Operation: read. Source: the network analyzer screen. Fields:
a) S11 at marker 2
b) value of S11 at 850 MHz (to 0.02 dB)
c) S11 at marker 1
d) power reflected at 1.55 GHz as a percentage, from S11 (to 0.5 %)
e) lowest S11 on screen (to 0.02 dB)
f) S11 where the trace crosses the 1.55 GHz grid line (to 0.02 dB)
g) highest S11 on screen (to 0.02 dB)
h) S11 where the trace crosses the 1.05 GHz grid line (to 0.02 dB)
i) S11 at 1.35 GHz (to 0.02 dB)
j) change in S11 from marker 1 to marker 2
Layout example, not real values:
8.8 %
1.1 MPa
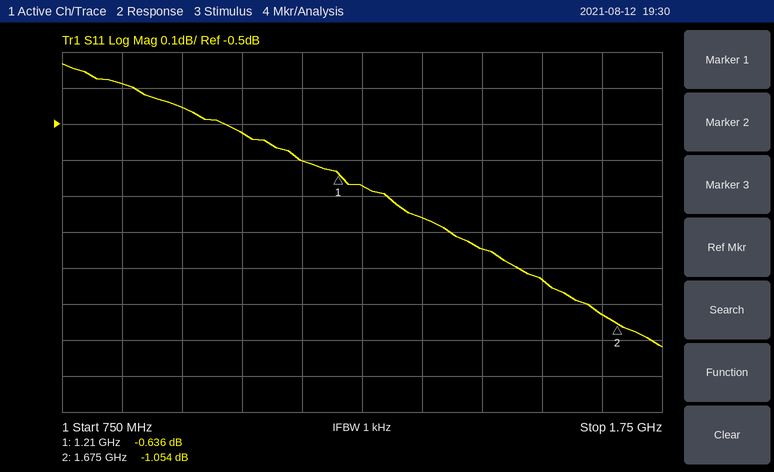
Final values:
-1.054 dB
-0.38 dB
-0.636 dB
80.5 %
-1.12 dB
-0.94 dB
-0.34 dB
-0.52 dB
-0.76 dB
-0.418 dB
